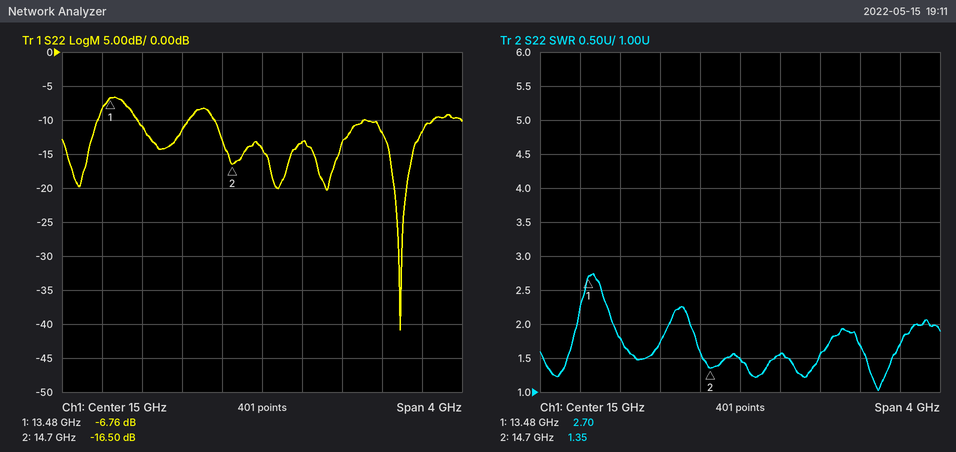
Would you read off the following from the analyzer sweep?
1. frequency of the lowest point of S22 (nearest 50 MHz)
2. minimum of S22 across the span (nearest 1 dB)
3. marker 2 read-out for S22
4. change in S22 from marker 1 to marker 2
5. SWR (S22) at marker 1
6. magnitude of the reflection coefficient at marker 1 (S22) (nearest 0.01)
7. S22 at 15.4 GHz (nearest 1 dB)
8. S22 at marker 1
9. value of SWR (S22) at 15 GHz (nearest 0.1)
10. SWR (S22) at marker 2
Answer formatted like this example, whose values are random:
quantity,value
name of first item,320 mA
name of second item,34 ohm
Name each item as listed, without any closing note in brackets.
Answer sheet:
quantity,value
frequency of the lowest point of S22,16.40 GHz
minimum of S22 across the span,-41 dB
marker 2 read-out for S22,-16.50 dB
change in S22 from marker 1 to marker 2,-9.74 dB
SWR (S22) at marker 1,2.70
magnitude of the reflection coefficient at marker 1 (S22),0.46
S22 at 15.4 GHz,-13 dB
S22 at marker 1,-6.76 dB
value of SWR (S22) at 15 GHz,1.5
SWR (S22) at marker 2,1.35
